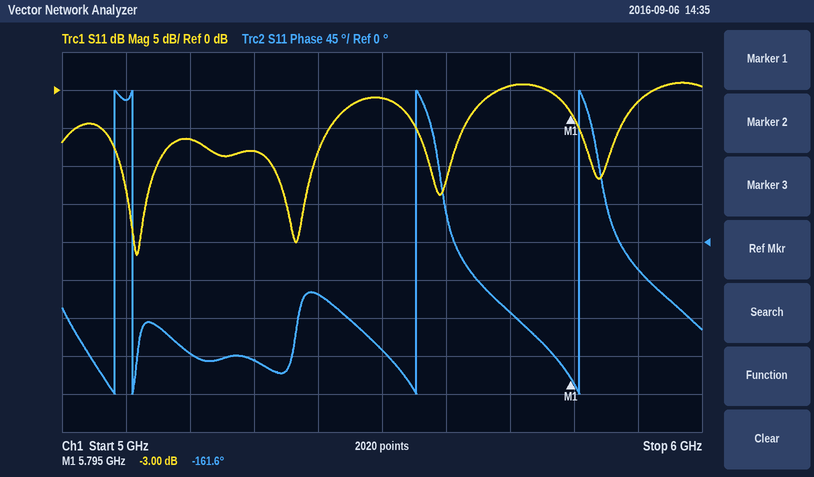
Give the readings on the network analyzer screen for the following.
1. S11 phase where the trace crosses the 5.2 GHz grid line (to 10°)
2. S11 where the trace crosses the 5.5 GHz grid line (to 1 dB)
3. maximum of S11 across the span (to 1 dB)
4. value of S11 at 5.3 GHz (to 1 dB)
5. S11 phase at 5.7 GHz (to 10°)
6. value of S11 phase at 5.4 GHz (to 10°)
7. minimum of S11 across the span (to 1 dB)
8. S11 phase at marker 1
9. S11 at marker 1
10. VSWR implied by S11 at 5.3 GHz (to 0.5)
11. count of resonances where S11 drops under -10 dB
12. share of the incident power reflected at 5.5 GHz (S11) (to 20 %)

-130°
-1 dB
1 dB
-8 dB
-80°
-60°
-22 dB
-161.6°
-3.00 dB
2.5
4
80 %
